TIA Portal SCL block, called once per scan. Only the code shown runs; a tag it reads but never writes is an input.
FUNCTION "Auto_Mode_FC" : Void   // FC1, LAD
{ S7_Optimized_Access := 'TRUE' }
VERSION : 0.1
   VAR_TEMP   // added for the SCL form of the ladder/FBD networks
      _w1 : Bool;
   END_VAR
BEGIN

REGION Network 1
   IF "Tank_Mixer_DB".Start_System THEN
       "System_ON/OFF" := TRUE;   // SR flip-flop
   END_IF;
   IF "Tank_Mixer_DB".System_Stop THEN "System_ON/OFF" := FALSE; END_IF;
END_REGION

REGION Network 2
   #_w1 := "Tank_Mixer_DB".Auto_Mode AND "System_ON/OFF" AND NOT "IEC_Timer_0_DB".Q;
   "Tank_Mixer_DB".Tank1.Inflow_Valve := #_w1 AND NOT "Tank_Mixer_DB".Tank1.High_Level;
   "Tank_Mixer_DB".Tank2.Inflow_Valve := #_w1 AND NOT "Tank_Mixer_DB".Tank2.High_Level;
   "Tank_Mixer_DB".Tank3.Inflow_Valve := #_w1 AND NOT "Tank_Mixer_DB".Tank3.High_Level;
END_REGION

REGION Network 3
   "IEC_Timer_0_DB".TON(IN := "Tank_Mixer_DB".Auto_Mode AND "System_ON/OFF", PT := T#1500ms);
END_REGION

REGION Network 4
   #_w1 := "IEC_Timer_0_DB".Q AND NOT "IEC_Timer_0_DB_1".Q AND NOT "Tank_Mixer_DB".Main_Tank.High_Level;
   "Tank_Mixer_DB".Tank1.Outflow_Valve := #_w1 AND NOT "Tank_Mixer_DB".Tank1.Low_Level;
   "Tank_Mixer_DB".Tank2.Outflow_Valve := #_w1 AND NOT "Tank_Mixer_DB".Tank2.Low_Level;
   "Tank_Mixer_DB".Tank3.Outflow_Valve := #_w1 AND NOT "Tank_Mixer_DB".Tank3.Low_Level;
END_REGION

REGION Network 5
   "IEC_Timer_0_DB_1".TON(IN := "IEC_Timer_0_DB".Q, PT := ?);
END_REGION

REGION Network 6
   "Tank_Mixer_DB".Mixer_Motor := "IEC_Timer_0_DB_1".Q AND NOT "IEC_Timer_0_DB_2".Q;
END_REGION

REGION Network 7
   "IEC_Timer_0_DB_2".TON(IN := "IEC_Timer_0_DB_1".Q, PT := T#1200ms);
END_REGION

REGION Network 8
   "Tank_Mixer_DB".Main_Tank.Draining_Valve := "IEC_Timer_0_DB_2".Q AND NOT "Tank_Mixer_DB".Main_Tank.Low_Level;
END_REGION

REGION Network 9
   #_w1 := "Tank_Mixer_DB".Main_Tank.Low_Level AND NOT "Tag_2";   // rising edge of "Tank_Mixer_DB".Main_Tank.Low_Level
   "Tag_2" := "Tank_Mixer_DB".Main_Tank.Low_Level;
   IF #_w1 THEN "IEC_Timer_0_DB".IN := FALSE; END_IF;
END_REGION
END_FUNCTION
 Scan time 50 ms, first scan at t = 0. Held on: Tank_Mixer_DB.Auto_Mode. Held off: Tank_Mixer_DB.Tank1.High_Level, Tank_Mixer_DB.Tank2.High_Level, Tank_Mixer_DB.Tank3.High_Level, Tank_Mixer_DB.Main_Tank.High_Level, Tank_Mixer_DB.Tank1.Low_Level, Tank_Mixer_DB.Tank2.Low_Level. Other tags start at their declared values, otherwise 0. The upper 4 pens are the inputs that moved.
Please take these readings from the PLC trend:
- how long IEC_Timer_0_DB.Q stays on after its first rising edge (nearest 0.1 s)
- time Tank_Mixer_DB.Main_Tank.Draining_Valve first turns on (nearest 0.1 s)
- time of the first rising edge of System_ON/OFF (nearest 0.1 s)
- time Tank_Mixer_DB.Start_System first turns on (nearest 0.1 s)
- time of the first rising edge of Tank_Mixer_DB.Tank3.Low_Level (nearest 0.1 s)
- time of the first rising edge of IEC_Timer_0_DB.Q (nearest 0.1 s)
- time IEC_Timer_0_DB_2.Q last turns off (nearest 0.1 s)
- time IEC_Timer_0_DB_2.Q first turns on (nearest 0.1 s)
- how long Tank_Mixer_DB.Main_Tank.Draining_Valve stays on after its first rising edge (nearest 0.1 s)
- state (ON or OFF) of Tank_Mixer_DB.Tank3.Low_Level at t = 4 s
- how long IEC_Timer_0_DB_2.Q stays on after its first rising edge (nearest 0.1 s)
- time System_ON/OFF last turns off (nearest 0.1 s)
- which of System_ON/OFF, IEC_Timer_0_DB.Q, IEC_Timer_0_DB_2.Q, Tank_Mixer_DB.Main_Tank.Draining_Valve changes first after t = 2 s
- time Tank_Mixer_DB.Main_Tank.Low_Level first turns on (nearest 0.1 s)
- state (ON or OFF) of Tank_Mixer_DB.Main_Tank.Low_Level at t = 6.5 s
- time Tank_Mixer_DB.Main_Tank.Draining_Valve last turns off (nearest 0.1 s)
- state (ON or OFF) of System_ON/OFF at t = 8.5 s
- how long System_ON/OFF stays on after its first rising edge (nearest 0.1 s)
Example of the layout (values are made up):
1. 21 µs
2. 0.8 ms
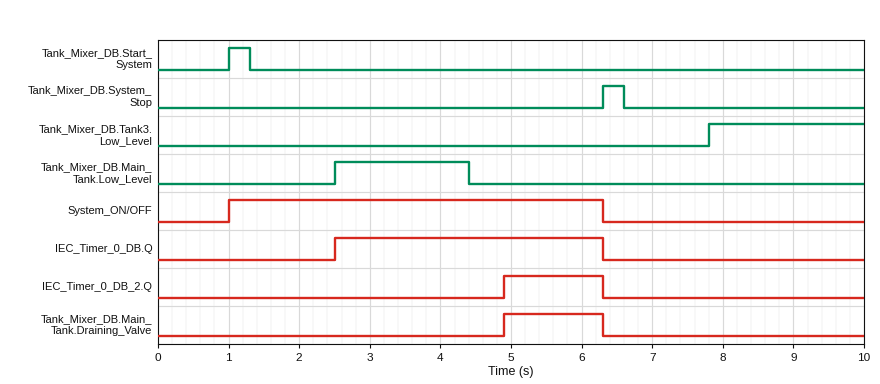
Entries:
1. 3.8 s
2. 4.9 s
3. 1.0 s
4. 1.0 s
5. 7.8 s
6. 2.5 s
7. 6.3 s
8. 4.9 s
9. 1.4 s
10. OFF
11. 1.4 s
12. 6.3 s
13. IEC_Timer_0_DB.Q
14. 2.5 s
15. OFF
16. 6.3 s
17. OFF
18. 5.3 s
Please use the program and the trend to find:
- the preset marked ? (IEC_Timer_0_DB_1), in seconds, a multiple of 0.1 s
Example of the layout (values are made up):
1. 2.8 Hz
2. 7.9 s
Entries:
1. 1.2 s
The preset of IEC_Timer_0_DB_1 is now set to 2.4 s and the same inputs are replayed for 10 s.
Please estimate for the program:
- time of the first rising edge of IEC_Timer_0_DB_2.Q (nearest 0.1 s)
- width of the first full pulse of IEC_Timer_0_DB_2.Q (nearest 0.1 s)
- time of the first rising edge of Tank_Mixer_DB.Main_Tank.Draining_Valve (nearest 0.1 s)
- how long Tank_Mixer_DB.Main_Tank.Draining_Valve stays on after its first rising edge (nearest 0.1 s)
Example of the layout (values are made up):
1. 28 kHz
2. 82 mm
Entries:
1. 6.1 s
2. 0.2 s
3. 6.1 s
4. 0.2 s
